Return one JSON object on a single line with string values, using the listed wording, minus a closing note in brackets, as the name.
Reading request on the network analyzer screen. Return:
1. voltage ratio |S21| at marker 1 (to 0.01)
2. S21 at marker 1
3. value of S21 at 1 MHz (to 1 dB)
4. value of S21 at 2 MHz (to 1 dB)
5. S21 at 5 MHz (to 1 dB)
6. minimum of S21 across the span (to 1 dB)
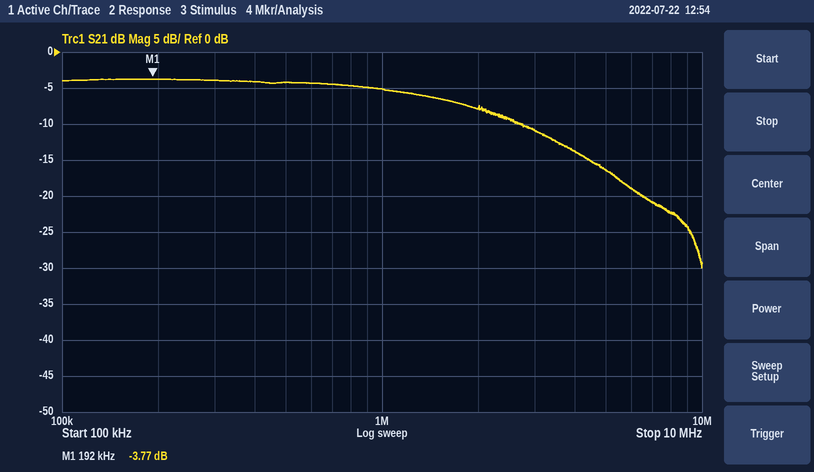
{"voltage ratio |S21| at marker 1": "0.65", "S21 at marker 1": "-3.77 dB", "value of S21 at 1 MHz": "-5 dB", "value of S21 at 2 MHz": "-8 dB", "S21 at 5 MHz": "-16 dB", "minimum of S21 across the span": "-30 dB"}
